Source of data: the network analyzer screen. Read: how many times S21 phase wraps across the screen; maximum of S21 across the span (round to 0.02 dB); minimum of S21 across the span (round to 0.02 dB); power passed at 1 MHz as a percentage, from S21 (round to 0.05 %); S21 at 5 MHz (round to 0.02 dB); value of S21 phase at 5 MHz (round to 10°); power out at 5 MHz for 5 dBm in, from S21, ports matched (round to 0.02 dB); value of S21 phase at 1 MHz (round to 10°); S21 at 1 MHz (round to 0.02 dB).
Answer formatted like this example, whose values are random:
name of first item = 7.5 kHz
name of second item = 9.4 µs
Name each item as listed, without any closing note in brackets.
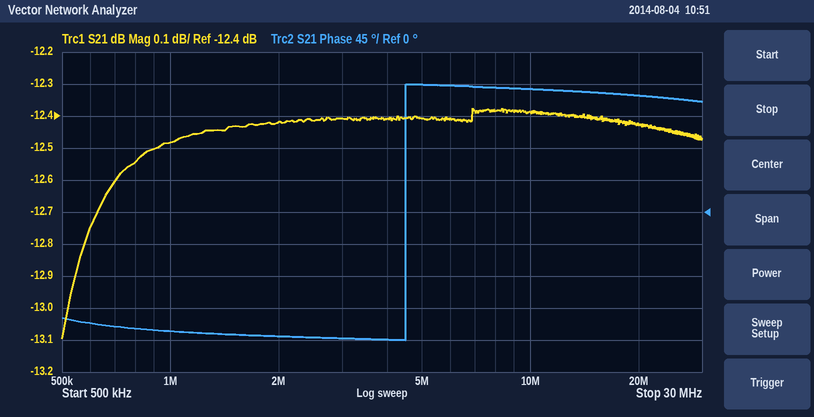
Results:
how many times S21 phase wraps across the screen = 1
maximum of S21 across the span = -12.38 dB
minimum of S21 across the span = -13.10 dB
power passed at 1 MHz as a percentage, from S21 = 5.65 %
S21 at 5 MHz = -12.40 dB
value of S21 phase at 5 MHz = 180°
power out at 5 MHz for 5 dBm in, from S21, ports matched = -7.40 dBm
value of S21 phase at 1 MHz = -170°
S21 at 1 MHz = -12.48 dB
